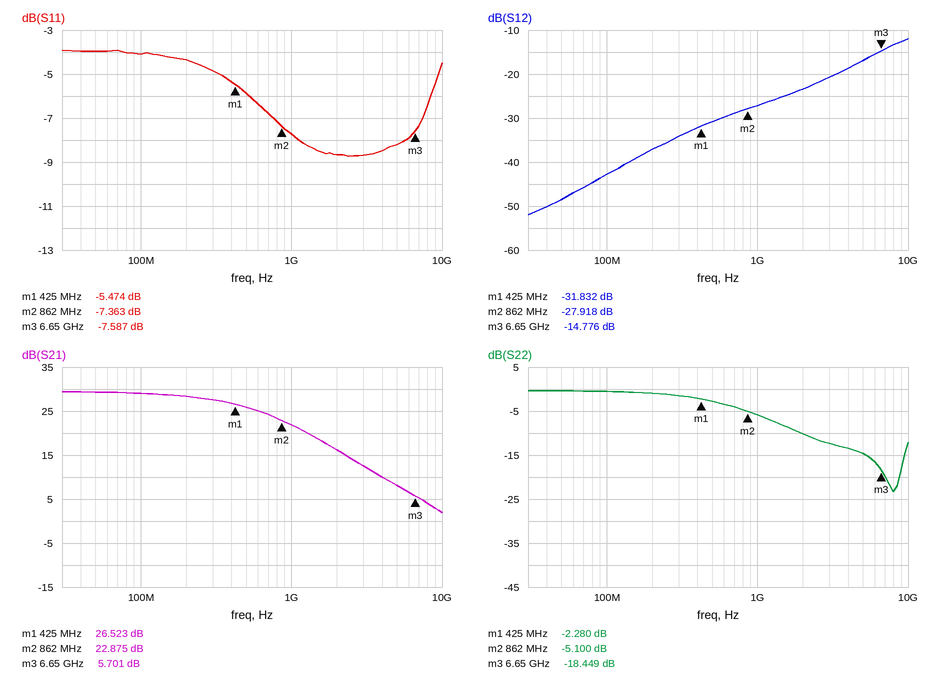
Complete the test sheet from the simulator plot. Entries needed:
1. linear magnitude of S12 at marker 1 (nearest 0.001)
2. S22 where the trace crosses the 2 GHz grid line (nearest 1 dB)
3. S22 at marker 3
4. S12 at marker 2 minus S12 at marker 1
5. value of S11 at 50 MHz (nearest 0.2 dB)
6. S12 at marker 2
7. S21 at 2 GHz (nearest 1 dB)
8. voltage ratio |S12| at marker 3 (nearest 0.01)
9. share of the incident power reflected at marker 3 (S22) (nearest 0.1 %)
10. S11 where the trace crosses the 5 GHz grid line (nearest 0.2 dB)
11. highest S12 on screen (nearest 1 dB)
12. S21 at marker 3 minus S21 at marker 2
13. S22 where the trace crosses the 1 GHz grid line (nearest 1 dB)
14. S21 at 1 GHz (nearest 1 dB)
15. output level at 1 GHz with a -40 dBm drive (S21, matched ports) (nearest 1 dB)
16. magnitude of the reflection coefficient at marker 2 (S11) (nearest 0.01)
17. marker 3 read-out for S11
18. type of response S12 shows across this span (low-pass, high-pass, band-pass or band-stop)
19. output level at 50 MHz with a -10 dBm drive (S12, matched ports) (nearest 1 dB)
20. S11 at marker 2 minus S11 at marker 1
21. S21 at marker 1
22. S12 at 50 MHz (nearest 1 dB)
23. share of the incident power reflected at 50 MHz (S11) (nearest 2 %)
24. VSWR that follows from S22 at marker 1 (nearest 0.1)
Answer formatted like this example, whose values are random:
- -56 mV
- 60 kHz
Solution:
- 0.026
- -10 dB
- -18.449 dB
- 3.914 dB
- -4.0 dB
- -27.918 dB
- 16 dB
- 0.18
- 1.4 %
- -8.2 dB
- -12 dB
- -17.174 dB
- -6 dB
- 22 dB
- -18 dBm
- 0.43
- -7.587 dB
- high-pass
- -59 dBm
- -1.889 dB
- 26.523 dB
- -49 dB
- 40 %
- 7.7
